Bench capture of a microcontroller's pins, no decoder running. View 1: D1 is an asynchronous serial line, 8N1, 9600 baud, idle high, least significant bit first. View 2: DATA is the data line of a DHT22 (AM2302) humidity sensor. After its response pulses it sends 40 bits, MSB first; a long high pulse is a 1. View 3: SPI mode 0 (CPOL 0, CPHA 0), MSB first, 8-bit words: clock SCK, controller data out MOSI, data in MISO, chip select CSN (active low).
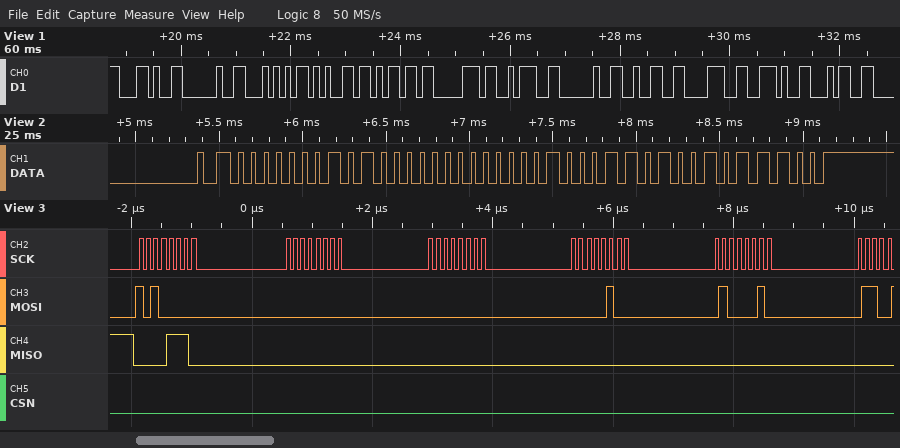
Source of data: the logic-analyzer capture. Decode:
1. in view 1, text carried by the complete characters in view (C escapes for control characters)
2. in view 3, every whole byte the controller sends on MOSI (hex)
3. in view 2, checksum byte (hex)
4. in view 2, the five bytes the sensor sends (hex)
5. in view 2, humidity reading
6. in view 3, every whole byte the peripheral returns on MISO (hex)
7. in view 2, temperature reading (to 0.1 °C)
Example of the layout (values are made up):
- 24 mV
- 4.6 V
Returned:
- ", Temp: 28.4"
- A0 00 00 04 42
- 0x5C
- 01 40 01 1A 5C
- 32.0 %
- 0E 00 00 00 00
- 28.2 °C
